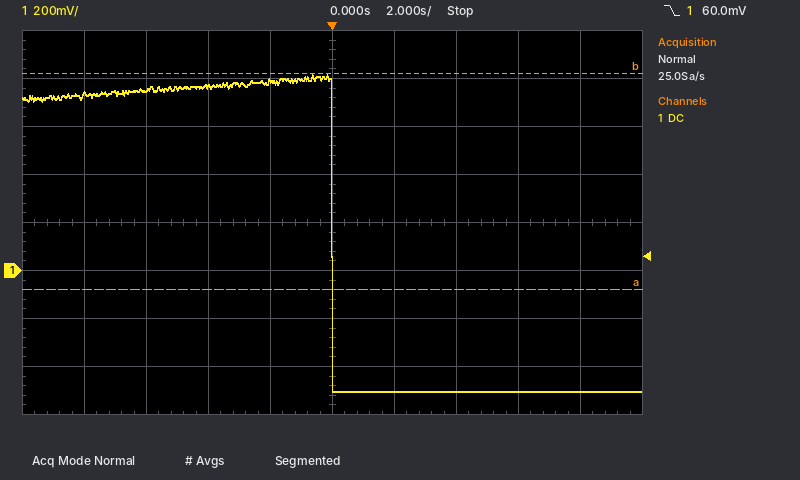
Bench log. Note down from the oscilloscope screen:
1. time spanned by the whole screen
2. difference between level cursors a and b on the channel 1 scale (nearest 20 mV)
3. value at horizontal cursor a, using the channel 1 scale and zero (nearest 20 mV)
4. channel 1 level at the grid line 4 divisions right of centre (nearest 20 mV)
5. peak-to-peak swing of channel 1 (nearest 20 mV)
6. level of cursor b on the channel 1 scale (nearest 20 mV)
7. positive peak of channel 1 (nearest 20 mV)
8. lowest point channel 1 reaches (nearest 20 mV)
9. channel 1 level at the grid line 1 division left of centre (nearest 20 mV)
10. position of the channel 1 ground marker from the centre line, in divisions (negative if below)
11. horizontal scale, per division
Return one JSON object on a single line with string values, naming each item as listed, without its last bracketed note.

{"time spanned by the whole screen": "20 s", "difference between level cursors a and b on the channel 1 scale": "900 mV", "value at horizontal cursor a, using the channel 1 scale and zero": "-80 mV", "channel 1 level at the grid line 4 divisions right of centre": "-500 mV", "peak-to-peak swing of channel 1": "1.32 V", "level of cursor b on the channel 1 scale": "820 mV", "positive peak of channel 1": "820 mV", "lowest point channel 1 reaches": "-500 mV", "channel 1 level at the grid line 1 division left of centre": "780 mV", "position of the channel 1 ground marker from the centre line, in divisions": "-1.0 div", "horizontal scale, per division": "2 s"}
